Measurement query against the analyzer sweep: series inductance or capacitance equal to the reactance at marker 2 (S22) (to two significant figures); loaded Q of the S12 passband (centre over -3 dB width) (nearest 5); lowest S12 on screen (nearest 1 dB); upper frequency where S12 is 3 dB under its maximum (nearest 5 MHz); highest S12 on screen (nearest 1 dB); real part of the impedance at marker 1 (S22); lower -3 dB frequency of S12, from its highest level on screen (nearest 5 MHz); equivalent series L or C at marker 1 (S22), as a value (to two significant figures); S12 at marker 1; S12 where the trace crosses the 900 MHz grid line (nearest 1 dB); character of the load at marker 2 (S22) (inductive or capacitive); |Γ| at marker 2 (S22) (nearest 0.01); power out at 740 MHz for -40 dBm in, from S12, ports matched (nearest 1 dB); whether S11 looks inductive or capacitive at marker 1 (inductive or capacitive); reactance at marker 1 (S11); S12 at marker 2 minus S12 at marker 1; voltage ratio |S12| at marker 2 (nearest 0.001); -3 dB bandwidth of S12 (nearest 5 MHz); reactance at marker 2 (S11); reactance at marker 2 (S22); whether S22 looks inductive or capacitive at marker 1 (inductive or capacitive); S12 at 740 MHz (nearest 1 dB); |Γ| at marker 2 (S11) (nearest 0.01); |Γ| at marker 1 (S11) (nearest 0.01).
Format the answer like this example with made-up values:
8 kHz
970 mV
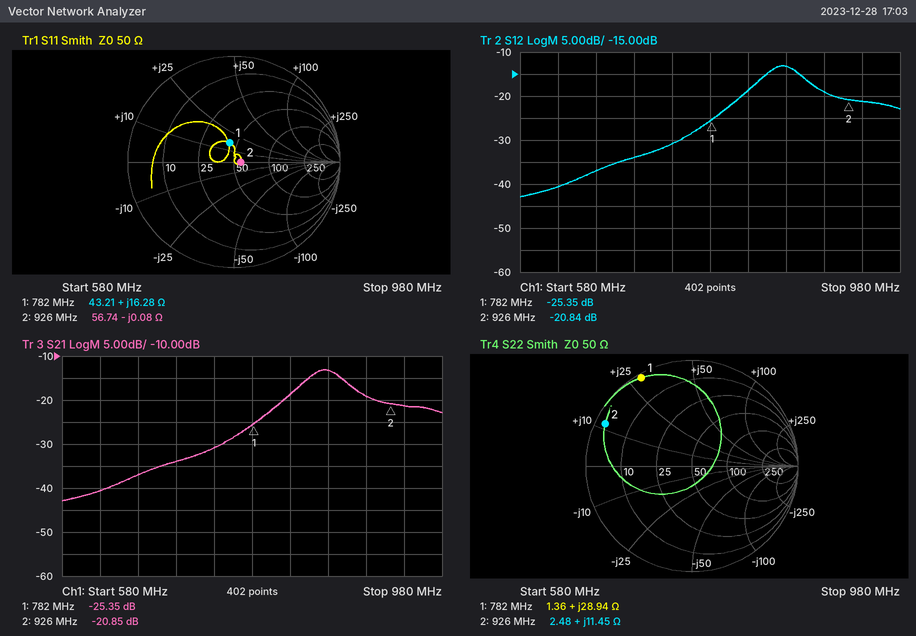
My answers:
2.0 nH
20
-43 dB
880 MHz
-13 dB
1.36 Ω
835 MHz
5.9 nH
-25.35 dB
-19 dB
inductive
0.91
-71 dBm
inductive
+16.28 Ω
4.51 dB
0.091
45 MHz
-0.08 Ω
+11.45 Ω
inductive
-31 dB
0.06
0.19
